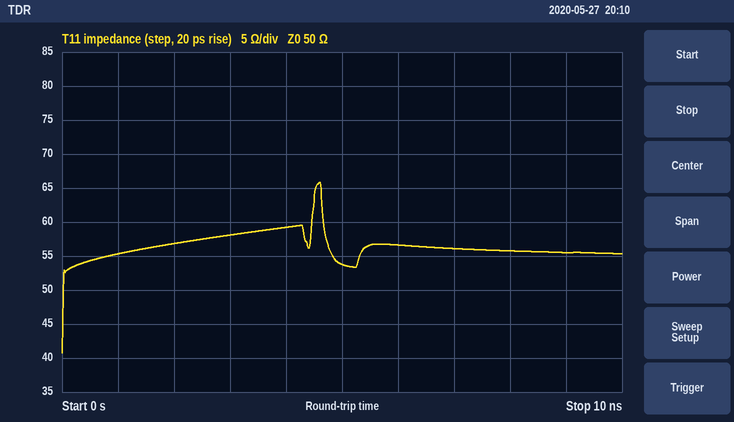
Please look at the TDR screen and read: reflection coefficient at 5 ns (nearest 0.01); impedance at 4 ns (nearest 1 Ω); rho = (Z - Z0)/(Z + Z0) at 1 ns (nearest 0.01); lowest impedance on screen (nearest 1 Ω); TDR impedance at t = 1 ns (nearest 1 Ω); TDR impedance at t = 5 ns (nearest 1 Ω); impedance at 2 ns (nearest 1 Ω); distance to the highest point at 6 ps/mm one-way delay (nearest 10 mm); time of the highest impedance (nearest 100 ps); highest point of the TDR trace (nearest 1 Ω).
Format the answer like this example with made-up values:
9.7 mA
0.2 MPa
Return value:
+0.04
59 Ω
+0.05
41 Ω
55 Ω
54 Ω
57 Ω
380 mm
4.6 ns
66 Ω
